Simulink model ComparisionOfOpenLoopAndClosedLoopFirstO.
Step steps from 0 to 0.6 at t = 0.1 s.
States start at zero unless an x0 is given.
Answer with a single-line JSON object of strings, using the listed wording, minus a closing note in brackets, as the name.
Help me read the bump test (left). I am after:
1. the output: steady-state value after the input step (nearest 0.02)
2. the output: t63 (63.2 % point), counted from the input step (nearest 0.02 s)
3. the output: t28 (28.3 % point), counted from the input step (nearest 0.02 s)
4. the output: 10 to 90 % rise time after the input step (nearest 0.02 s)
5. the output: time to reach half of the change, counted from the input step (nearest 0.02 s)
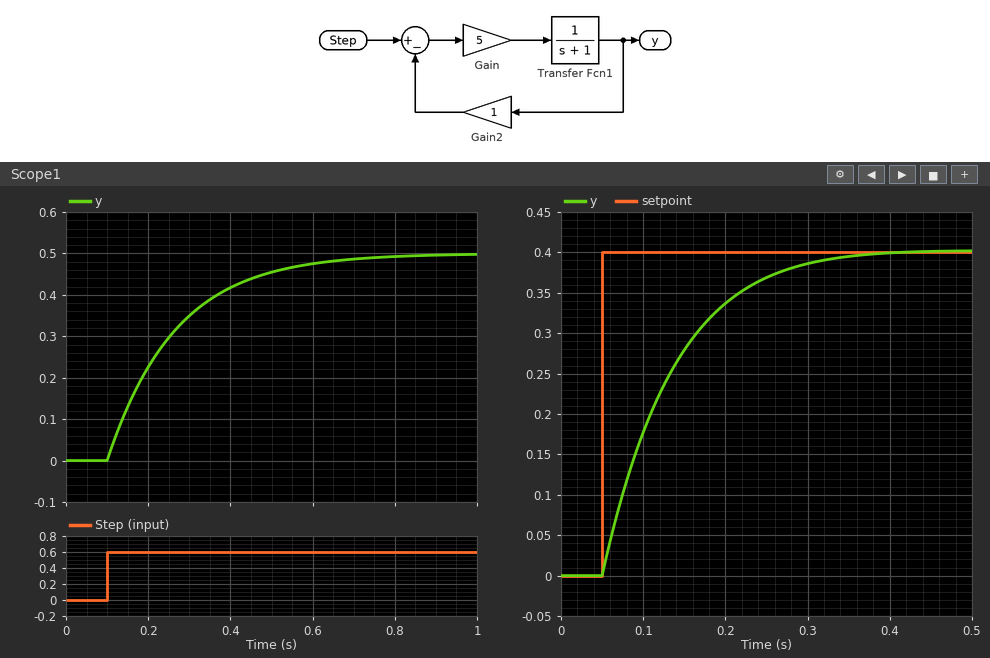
{"the output: steady-state value after the input step": "0.50", "the output: t63 (63.2 % point), counted from the input step": "0.16 s", "the output: t28 (28.3 % point), counted from the input step": "0.06 s", "the output: 10 to 90 % rise time after the input step": "0.36 s", "the output: time to reach half of the change, counted from the input step": "0.12 s"}
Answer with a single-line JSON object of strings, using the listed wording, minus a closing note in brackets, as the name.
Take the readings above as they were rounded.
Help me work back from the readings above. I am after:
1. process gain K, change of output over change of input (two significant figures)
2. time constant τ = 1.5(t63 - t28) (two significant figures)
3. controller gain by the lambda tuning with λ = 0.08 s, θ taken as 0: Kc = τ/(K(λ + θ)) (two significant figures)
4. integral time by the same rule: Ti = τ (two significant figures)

{"process gain K, change of output over change of input": "0.83", "time constant τ = 1.5(t63 - t28)": "0.15 s", "controller gain by the lambda tuning with λ = 0.08 s, θ taken as 0: Kc = τ/(K(λ + θ))": "2.3", "integral time by the same rule: Ti = τ": "0.15 s"}
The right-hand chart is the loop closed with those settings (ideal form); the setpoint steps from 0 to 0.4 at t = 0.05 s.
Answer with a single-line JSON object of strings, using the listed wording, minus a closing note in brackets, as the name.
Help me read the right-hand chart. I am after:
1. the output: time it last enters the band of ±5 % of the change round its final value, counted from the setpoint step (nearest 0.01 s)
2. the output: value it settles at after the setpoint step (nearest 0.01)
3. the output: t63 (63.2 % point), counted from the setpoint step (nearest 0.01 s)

{"the output: time it last enters the band of ±5 % of the change round its final value, counted from the setpoint step": "0.23 s", "the output: value it settles at after the setpoint step": "0.40", "the output: t63 (63.2 % point), counted from the setpoint step": "0.08 s"}
